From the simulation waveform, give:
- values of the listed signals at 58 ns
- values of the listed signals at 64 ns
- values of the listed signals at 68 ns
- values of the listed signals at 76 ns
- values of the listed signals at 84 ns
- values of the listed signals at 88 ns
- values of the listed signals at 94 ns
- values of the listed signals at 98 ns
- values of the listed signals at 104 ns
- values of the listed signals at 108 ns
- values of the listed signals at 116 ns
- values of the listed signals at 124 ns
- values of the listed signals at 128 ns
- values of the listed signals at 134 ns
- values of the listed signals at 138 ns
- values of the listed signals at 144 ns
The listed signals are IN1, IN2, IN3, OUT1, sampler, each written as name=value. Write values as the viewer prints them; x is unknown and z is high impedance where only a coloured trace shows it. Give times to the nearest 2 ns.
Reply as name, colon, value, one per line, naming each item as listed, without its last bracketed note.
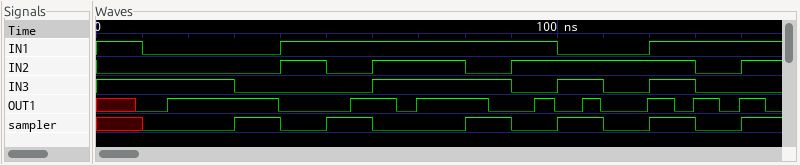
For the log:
values of the listed signals at 58 ns: IN1=1, IN2=0, IN3=0, OUT1=1, sampler=1
values of the listed signals at 64 ns: IN1=1, IN2=1, IN3=1, OUT1=1, sampler=0
values of the listed signals at 68 ns: IN1=1, IN2=1, IN3=1, OUT1=0, sampler=0
values of the listed signals at 76 ns: IN1=1, IN2=1, IN3=1, OUT1=1, sampler=0
values of the listed signals at 84 ns: IN1=1, IN2=0, IN3=1, OUT1=1, sampler=1
values of the listed signals at 88 ns: IN1=1, IN2=0, IN3=1, OUT1=0, sampler=1
values of the listed signals at 94 ns: IN1=1, IN2=1, IN3=0, OUT1=0, sampler=0
values of the listed signals at 98 ns: IN1=1, IN2=1, IN3=0, OUT1=1, sampler=0
values of the listed signals at 104 ns: IN1=0, IN2=1, IN3=1, OUT1=0, sampler=1
values of the listed signals at 108 ns: IN1=0, IN2=1, IN3=1, OUT1=1, sampler=1
values of the listed signals at 116 ns: IN1=0, IN2=1, IN3=0, OUT1=0, sampler=0
values of the listed signals at 124 ns: IN1=1, IN2=1, IN3=1, OUT1=1, sampler=1
values of the listed signals at 128 ns: IN1=1, IN2=1, IN3=1, OUT1=0, sampler=1
values of the listed signals at 134 ns: IN1=1, IN2=0, IN3=0, OUT1=1, sampler=0
values of the listed signals at 138 ns: IN1=1, IN2=0, IN3=0, OUT1=0, sampler=0
values of the listed signals at 144 ns: IN1=1, IN2=1, IN3=0, OUT1=1, sampler=1
